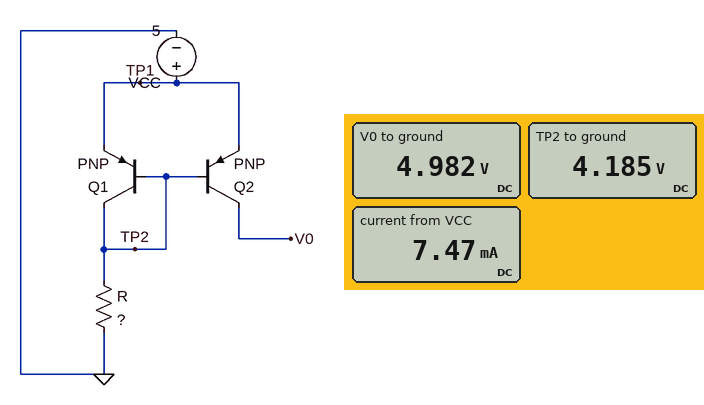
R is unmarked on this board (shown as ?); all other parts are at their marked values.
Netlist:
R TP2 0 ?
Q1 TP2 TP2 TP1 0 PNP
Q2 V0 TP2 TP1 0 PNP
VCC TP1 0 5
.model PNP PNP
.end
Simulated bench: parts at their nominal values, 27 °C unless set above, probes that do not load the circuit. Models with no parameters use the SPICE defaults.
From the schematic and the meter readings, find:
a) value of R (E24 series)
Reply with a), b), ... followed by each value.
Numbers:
a) 560 Ω
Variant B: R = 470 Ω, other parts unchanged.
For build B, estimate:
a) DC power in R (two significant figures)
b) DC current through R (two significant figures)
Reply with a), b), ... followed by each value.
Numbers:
a) 37 mW
b) 8.9 mA
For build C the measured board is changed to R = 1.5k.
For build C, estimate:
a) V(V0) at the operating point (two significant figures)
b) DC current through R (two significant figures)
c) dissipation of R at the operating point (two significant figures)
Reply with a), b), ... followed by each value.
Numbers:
a) 5.0 V
b) 2.8 mA
c) 12 mW
